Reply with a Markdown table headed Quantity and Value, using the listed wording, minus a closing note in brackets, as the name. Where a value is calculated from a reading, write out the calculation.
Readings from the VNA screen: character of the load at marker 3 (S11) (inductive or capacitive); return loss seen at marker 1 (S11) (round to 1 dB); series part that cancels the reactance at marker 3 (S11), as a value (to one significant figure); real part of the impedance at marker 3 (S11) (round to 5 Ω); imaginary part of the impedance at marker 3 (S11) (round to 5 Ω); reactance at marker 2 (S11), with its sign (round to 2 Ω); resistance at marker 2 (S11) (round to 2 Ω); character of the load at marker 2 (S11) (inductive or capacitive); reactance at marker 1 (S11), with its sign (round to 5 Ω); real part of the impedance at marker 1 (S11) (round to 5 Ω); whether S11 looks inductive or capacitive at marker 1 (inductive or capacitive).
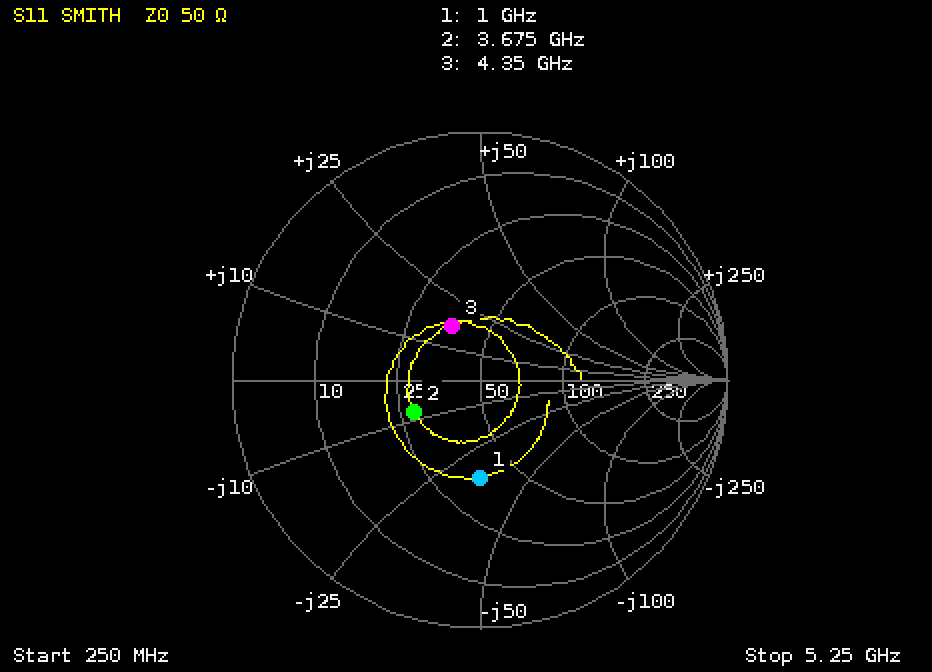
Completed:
| Quantity | Value |
|---|---|
| character of the load at marker 3 (S11) | inductive |
| return loss seen at marker 1 (S11) | 8 dB |
| series part that cancels the reactance at marker 3 (S11), as a value | C = 1/(2π × 4.35 GHz × 15 Ω) ≈ 2 pF |
| real part of the impedance at marker 3 (S11) | 35 Ω |
| imaginary part of the impedance at marker 3 (S11) | +15 Ω |
| reactance at marker 2 (S11), with its sign | -8 Ω |
| resistance at marker 2 (S11) | 28 Ω |
| character of the load at marker 2 (S11) | capacitive |
| reactance at marker 1 (S11), with its sign | -35 Ω |
| real part of the impedance at marker 1 (S11) | 35 Ω |
| whether S11 looks inductive or capacitive at marker 1 | capacitive |
